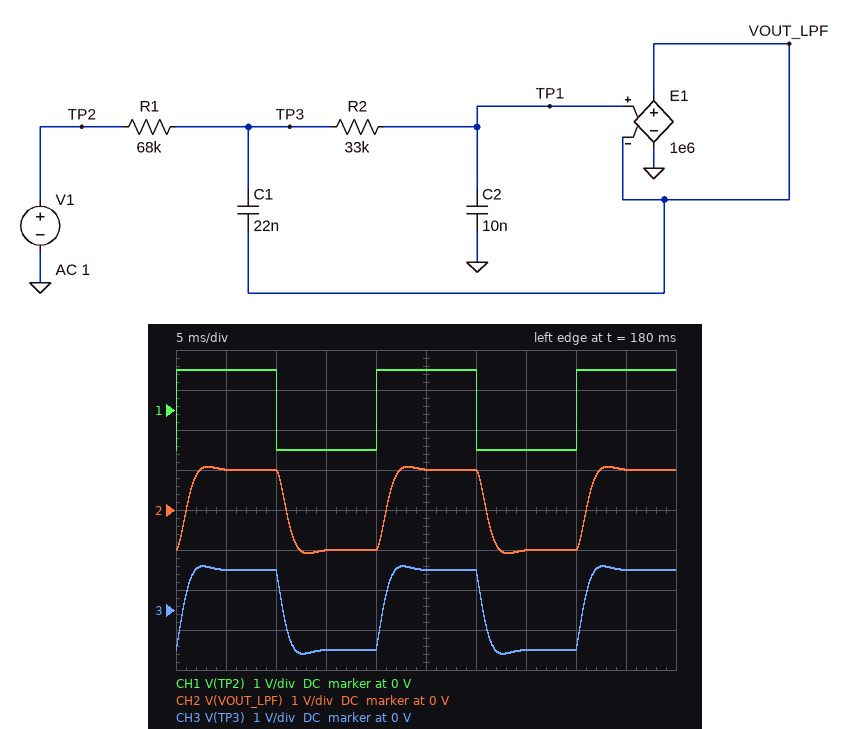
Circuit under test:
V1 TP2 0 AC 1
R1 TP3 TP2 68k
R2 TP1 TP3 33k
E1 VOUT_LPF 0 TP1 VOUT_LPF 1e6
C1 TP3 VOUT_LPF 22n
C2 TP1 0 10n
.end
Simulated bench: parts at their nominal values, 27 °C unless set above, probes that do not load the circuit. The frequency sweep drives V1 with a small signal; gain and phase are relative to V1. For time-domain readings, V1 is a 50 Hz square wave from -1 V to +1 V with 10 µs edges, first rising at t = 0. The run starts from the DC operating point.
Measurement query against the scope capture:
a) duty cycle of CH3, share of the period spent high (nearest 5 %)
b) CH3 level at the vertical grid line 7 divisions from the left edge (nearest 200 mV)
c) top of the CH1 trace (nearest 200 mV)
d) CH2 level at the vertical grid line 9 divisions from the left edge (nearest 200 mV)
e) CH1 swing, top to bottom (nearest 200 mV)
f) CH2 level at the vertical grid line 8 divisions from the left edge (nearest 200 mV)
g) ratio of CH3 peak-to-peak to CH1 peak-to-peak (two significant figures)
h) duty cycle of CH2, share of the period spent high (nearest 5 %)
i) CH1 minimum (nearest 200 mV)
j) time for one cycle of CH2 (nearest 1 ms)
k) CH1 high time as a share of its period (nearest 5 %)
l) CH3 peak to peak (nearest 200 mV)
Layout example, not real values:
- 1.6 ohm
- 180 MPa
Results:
- 50 %
- -1.0 V
- 1.0 V
- 1.0 V
- 2.0 V
- -1.0 V
- 1.1
- 50 %
- -1.0 V
- 20 ms
- 50 %
- 2.2 V
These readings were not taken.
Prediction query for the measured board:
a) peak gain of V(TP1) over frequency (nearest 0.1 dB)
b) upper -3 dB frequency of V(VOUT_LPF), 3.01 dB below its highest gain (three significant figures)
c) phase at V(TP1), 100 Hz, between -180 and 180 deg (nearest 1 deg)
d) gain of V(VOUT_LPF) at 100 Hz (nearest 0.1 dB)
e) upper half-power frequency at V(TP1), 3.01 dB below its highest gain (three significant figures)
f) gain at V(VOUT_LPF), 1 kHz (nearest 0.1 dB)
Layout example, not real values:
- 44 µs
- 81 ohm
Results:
- 0 dB
- 223 Hz
- -38 deg
- -0.2 dB
- 223 Hz
- -25.8 dB
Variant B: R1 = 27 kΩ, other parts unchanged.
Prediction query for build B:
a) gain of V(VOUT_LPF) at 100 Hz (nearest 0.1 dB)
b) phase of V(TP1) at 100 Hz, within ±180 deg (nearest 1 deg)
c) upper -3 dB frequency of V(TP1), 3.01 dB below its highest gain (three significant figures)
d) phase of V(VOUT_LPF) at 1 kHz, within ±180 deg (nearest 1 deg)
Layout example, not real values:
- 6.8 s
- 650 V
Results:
- 0 dB
- -22 deg
- 373 Hz
- -151 deg
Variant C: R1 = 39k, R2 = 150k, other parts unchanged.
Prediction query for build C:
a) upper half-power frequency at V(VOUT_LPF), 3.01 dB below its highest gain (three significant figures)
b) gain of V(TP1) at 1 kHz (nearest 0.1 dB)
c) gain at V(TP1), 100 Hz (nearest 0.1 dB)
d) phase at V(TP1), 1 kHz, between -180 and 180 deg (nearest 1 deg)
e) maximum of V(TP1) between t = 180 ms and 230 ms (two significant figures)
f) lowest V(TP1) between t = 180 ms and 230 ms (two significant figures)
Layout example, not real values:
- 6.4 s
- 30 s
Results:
- 116 Hz
- -34.2 dB
- -2.2 dB
- -167 deg
- 1.0 V
- -1.0 V
